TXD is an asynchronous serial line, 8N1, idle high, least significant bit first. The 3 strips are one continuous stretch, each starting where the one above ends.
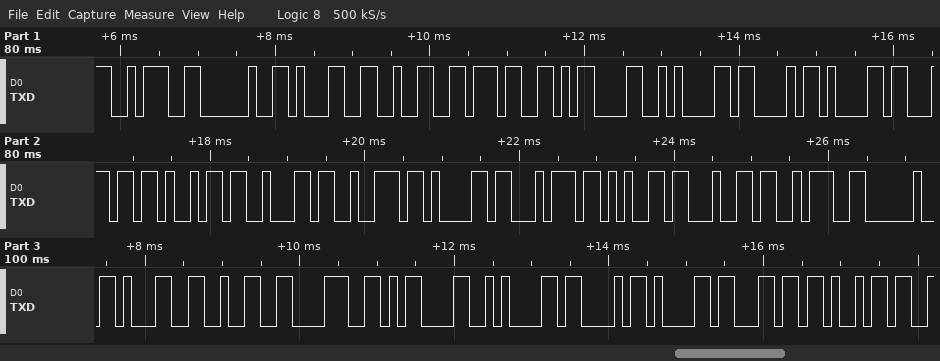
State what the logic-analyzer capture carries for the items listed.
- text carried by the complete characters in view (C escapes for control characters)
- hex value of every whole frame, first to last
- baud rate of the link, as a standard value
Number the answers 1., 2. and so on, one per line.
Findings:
1. ": 127\r\nCalibrated: 128\r\nCali"
2. 3A 20 31 32 37 0D 0A 43 61 6C 69 62 72 61 74 65 64 3A 20 31 32 38 0D 0A 43 61 6C 69
3. 9600 baud
